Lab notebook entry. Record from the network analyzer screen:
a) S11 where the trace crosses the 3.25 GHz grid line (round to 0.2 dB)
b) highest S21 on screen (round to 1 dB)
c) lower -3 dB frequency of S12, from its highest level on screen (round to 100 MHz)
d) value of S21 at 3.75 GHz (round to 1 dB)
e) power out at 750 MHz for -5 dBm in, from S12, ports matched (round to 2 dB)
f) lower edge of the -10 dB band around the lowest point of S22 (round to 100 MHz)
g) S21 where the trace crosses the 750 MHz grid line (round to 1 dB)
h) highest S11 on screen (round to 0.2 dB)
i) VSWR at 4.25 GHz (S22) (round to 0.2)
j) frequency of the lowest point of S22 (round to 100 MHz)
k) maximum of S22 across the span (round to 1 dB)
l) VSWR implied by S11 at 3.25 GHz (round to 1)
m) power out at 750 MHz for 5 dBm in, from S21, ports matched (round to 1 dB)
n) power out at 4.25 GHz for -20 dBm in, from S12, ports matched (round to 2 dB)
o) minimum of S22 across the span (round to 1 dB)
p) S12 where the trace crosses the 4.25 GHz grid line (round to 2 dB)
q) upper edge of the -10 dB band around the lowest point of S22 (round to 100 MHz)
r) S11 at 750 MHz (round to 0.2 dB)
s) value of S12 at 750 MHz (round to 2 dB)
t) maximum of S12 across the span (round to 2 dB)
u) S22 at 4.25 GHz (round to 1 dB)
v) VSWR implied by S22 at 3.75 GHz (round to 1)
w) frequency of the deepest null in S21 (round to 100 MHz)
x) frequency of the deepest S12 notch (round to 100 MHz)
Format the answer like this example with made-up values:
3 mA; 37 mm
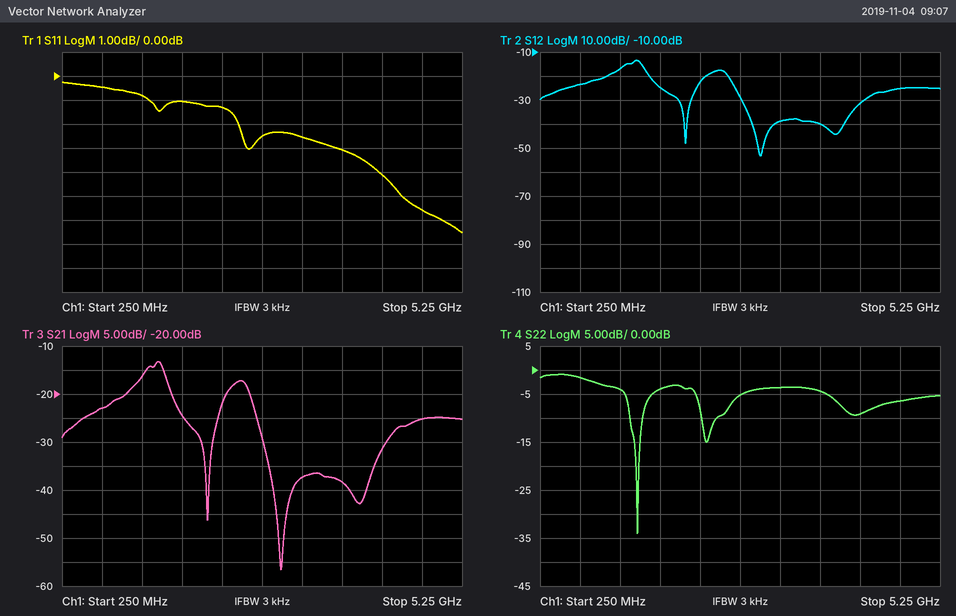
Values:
-2.6 dB; -13 dB; 1.3 GHz; -38 dB; -28 dBm; 1.4 GHz; -23 dB; -0.2 dB; 2.0; 1.5 GHz; -1 dB; 7; -18 dBm; -52 dBm; -34 dB; -32 dB; 1.5 GHz; -0.4 dB; -24 dB; -14 dB; -9 dB; 4; 3.0 GHz; 3.0 GHz
